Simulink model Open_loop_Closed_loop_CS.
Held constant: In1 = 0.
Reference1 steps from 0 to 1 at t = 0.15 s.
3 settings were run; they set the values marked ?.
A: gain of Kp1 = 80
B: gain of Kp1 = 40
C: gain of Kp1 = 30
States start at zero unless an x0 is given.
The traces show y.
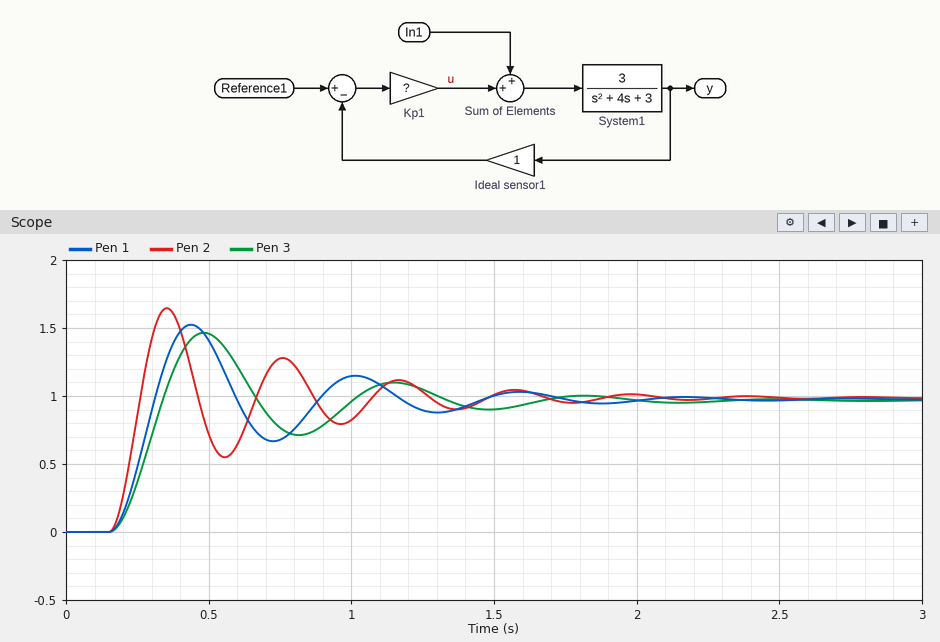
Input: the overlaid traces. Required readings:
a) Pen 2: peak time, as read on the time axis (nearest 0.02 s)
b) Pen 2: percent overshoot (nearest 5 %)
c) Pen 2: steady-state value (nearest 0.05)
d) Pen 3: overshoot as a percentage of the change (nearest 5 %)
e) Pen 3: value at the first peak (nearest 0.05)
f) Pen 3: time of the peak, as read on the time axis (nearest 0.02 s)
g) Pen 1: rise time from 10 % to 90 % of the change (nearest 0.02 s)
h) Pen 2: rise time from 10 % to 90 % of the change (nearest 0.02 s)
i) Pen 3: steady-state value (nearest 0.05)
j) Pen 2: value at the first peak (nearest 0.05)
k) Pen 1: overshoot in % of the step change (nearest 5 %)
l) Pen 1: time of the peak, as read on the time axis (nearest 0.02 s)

0.36 s
65 %
1.00
50 %
1.45
0.48 s
0.10 s
0.08 s
0.95
1.65
55 %
0.44 s
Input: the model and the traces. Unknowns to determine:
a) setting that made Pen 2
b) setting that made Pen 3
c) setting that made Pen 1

A
C
B
